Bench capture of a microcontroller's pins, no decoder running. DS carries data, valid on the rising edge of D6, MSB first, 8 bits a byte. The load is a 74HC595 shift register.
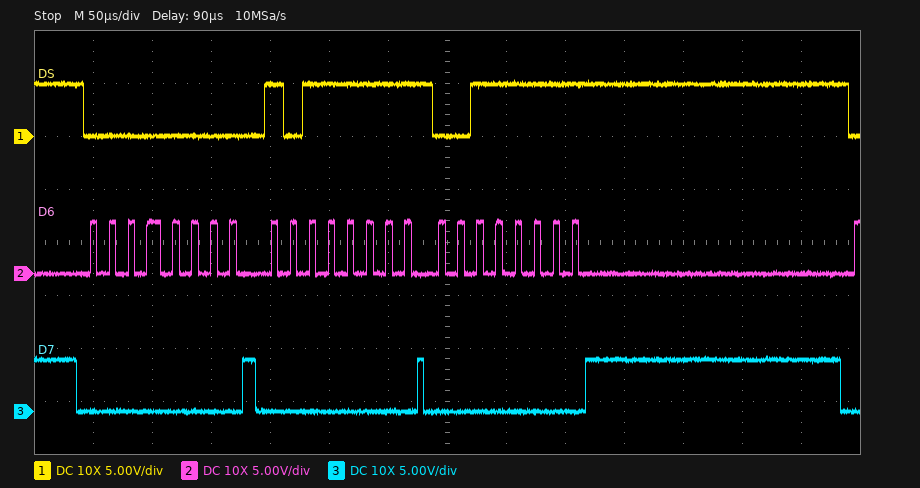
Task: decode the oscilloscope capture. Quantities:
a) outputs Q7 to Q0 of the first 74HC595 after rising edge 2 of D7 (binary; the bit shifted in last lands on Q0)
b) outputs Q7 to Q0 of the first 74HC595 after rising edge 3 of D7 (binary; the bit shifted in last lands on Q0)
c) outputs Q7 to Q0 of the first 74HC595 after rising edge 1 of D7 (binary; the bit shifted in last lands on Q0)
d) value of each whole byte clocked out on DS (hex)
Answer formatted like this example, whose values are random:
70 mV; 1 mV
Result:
10111111; 00111111; 00000000; 0x00 0xBF 0x3F
